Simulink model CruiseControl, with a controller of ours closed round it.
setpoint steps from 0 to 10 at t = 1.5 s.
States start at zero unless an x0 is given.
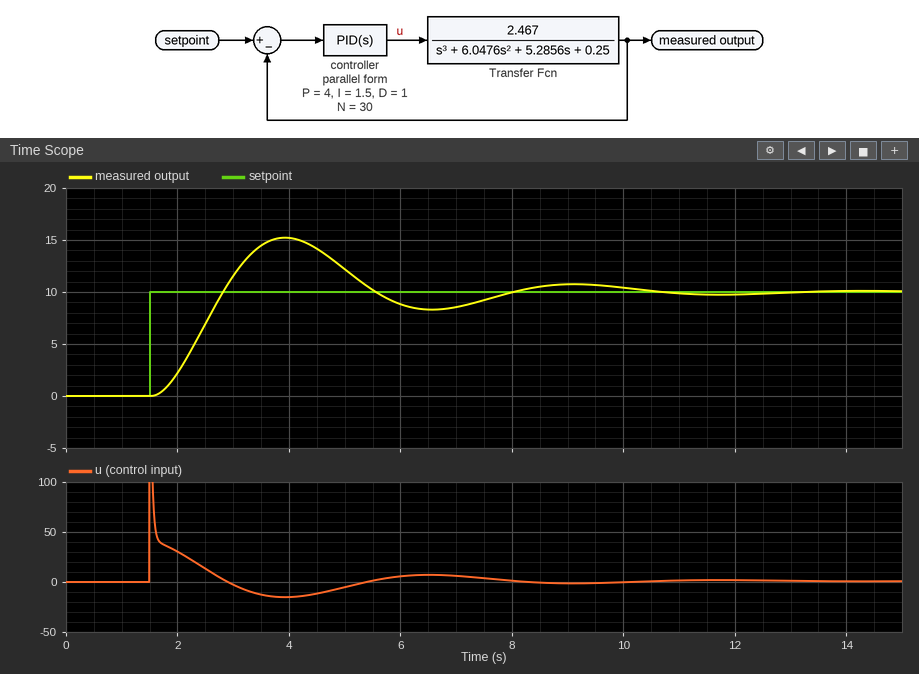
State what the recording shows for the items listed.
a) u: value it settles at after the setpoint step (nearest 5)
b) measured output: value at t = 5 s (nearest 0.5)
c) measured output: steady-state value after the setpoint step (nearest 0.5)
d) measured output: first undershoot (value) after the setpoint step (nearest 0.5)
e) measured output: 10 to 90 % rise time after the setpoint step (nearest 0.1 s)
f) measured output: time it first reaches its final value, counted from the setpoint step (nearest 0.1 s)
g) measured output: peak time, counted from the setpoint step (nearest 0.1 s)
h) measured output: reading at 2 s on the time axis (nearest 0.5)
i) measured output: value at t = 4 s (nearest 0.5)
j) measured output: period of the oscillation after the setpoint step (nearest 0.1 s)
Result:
0
12.0
10.0
8.5
0.9 s
1.3 s
2.4 s
2.0
15.0
5.2 s
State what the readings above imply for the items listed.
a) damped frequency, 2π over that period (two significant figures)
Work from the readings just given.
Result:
1.2 rad/s
